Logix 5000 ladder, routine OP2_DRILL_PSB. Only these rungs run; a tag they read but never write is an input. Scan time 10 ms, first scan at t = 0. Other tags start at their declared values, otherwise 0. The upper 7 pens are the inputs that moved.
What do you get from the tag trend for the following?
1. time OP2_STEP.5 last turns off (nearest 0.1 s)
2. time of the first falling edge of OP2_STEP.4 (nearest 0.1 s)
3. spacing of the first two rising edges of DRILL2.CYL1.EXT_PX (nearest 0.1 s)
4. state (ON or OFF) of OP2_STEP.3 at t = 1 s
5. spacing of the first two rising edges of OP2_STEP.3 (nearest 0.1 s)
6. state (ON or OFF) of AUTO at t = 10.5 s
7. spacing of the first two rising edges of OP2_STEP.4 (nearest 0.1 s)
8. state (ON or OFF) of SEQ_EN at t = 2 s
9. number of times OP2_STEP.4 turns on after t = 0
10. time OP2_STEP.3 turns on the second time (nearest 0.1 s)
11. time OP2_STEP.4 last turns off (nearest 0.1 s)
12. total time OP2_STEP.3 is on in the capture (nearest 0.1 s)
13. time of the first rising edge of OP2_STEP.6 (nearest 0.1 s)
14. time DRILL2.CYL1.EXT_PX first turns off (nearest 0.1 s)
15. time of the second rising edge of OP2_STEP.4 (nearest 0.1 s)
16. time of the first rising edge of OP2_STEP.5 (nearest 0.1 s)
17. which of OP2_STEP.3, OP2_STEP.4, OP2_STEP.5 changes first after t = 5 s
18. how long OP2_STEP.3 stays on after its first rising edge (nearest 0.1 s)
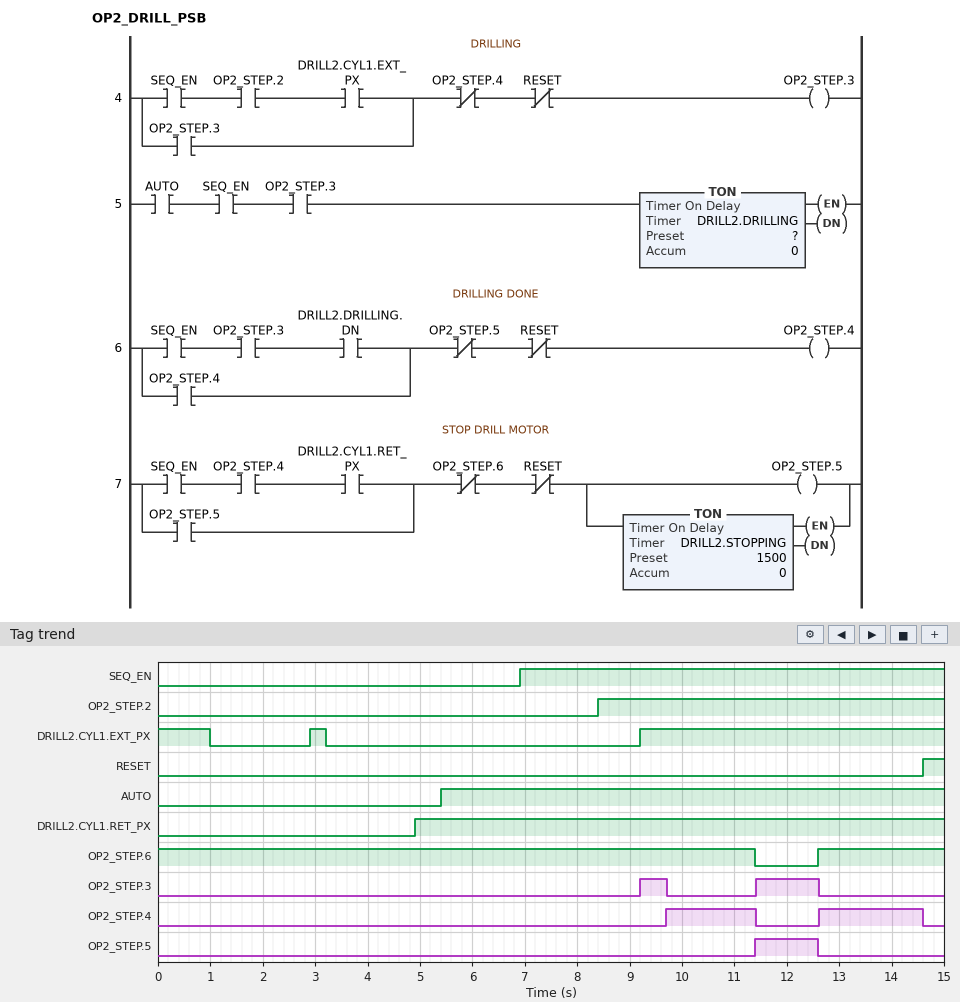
12.6 s
11.4 s
6.3 s
OFF
2.2 s
ON
2.9 s
OFF
2
11.4 s
14.6 s
1.7 s
12.6 s
1.0 s
12.6 s
11.4 s
OP2_STEP.3
0.5 s
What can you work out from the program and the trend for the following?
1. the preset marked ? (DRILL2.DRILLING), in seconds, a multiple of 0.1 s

0.5 s
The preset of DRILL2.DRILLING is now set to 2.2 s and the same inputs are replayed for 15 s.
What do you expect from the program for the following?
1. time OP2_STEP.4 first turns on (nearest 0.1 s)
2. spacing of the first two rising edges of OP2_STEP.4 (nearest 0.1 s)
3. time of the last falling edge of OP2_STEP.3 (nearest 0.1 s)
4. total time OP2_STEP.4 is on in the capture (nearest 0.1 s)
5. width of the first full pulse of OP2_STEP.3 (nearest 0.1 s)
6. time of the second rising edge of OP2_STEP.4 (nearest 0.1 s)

11.4 s
2.2 s
13.6 s
1.0 s
2.2 s
13.6 s
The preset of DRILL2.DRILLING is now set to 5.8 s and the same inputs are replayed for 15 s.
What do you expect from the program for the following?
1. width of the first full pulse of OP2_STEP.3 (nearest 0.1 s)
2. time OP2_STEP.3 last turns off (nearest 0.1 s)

5.4 s
14.6 s
